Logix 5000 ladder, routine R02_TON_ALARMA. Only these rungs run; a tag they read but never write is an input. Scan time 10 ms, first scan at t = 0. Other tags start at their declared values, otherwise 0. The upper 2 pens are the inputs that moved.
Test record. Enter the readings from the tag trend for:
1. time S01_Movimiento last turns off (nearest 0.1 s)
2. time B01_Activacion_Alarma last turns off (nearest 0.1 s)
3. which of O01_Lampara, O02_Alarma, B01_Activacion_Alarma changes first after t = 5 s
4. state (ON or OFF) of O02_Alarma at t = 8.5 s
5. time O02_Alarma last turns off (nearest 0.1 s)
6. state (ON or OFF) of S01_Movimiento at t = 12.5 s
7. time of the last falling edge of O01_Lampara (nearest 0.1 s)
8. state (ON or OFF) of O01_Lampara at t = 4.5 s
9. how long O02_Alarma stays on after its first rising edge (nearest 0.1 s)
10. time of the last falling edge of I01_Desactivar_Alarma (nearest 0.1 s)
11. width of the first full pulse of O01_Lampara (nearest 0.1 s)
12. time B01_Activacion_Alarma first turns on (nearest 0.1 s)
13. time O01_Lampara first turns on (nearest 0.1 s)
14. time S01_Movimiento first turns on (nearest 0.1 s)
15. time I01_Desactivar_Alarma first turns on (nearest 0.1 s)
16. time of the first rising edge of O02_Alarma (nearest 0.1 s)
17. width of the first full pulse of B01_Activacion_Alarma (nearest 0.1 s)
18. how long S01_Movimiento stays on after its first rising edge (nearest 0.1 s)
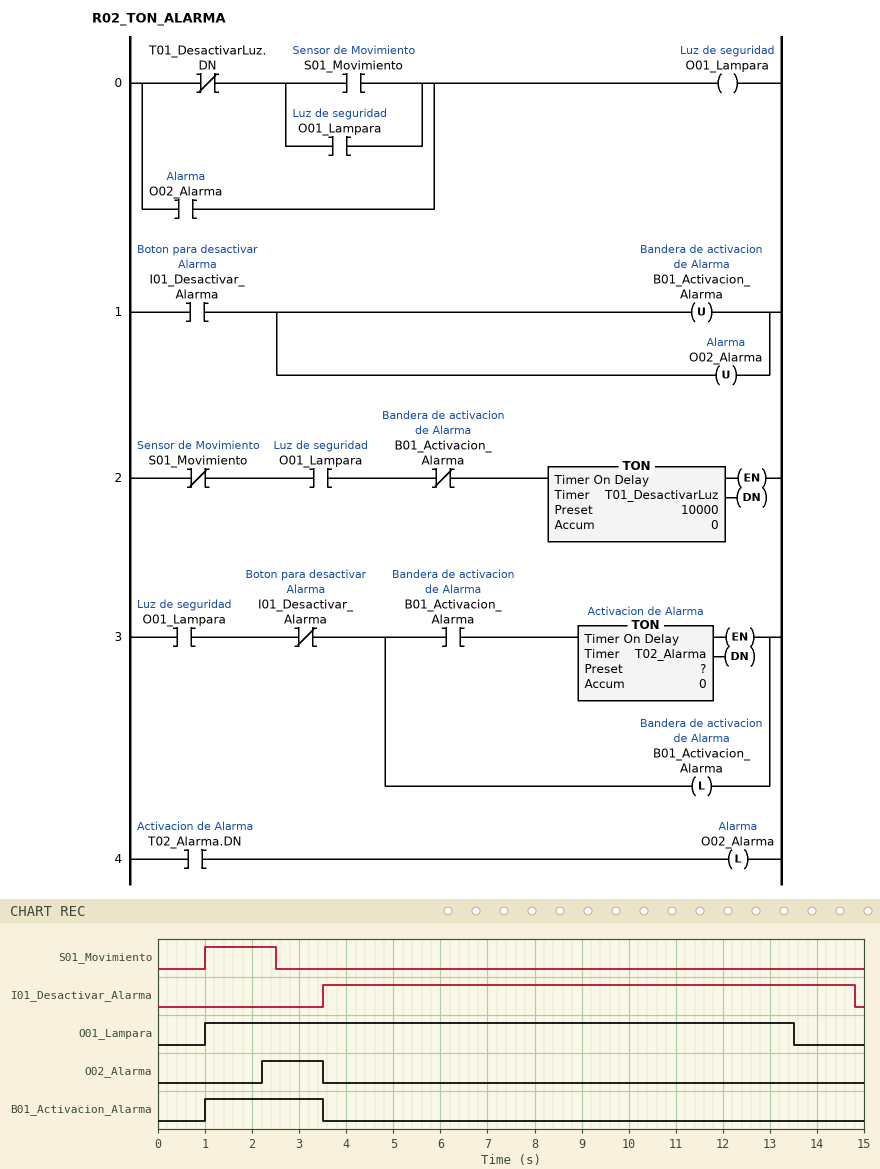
2.5 s
3.5 s
O01_Lampara
OFF
3.5 s
OFF
13.5 s
ON
1.3 s
14.8 s
12.5 s
1.0 s
1.0 s
1.0 s
3.5 s
2.2 s
2.5 s
1.5 s
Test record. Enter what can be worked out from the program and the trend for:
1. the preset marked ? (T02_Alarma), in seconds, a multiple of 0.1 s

1.2 s
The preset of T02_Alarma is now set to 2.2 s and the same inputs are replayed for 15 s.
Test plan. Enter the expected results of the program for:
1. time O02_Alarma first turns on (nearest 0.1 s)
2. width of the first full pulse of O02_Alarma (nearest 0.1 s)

3.2 s
0.3 s
